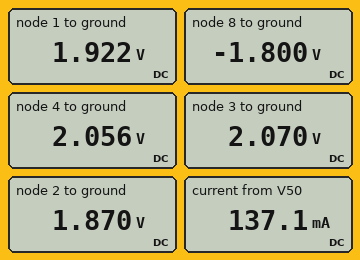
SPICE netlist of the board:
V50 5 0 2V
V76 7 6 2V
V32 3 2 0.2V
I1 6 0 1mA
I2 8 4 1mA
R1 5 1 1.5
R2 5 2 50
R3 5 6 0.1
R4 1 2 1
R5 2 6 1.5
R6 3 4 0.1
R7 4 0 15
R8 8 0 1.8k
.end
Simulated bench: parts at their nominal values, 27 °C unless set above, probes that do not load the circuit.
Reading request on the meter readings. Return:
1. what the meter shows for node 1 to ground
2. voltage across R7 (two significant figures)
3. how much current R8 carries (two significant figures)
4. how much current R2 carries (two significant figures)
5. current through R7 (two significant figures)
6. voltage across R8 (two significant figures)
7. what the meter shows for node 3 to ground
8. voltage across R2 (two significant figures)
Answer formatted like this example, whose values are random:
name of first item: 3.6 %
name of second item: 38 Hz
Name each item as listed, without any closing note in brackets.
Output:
what the meter shows for node 1 to ground: 1.922 V
voltage across R7: 2.1 V
how much current R8 carries: 1.0 mA
how much current R2 carries: 2.6 mA
current through R7: 140 mA
voltage across R8: 1.8 V
what the meter shows for node 3 to ground: 2.070 V
voltage across R2: 130 mV
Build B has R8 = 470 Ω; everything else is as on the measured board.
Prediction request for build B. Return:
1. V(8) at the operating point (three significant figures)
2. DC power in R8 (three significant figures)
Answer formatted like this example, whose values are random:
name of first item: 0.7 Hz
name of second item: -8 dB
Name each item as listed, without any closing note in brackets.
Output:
V(8) at the operating point: -470 mV
DC power in R8: 470 µW
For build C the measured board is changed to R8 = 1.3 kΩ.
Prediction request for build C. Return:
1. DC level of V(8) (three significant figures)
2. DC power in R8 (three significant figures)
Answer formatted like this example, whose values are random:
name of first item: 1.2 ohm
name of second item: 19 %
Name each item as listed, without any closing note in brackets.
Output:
DC level of V(8): -1.30 V
DC power in R8: 1.30 mW
